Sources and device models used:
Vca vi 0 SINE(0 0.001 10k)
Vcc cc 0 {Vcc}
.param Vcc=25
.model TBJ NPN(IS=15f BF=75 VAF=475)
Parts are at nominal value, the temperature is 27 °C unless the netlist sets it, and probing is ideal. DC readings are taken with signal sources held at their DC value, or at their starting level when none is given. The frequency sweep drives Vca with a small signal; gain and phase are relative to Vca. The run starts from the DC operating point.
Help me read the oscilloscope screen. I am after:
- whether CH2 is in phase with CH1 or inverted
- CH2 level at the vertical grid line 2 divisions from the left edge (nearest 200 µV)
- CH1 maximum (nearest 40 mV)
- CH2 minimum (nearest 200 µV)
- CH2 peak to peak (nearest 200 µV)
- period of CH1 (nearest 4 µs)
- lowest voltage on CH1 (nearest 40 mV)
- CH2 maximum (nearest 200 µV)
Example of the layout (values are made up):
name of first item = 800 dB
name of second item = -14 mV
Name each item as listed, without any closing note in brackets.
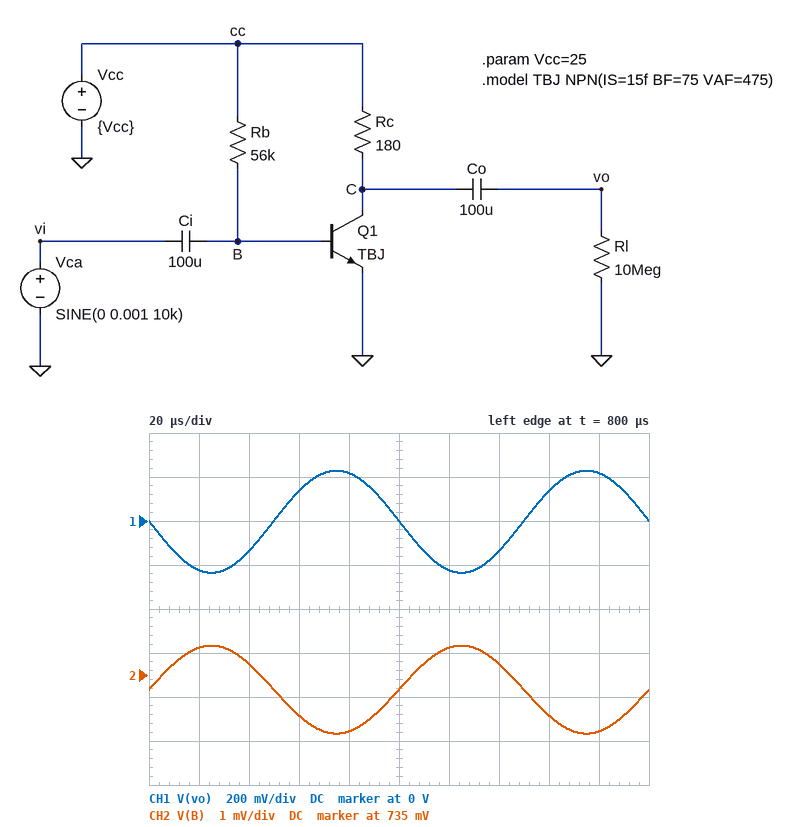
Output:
whether CH2 is in phase with CH1 or inverted = inverted
CH2 level at the vertical grid line 2 divisions from the left edge = 735.2 mV
CH1 maximum = 240 mV
CH2 minimum = 733.6 mV
CH2 peak to peak = 2.0 mV
period of CH1 = 100 µs
lowest voltage on CH1 = -240 mV
CH2 maximum = 735.6 mV
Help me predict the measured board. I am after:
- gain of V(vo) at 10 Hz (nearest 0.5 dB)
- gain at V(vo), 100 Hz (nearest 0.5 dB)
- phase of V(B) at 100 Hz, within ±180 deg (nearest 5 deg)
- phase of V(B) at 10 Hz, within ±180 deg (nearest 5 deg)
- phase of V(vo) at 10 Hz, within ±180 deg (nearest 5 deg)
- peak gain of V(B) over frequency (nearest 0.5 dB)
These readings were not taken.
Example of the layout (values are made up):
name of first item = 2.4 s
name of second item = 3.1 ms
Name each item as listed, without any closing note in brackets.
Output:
gain of V(vo) at 10 Hz = 38.0 dB
gain at V(vo), 100 Hz = 47.0 dB
phase of V(B) at 100 Hz, within ±180 deg = 15 deg
phase of V(B) at 10 Hz, within ±180 deg = 70 deg
phase of V(vo) at 10 Hz, within ±180 deg = -110 deg
peak gain of V(B) over frequency = 0 dB
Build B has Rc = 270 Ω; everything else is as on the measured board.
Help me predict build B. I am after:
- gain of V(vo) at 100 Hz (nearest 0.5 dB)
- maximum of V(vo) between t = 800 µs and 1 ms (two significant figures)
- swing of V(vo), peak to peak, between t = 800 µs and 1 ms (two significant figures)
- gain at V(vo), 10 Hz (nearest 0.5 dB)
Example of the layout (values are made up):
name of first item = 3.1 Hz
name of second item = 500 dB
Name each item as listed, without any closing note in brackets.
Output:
gain of V(vo) at 100 Hz = 50.5 dB
maximum of V(vo) between t = 800 µs and 1 ms = 340 mV
swing of V(vo), peak to peak, between t = 800 µs and 1 ms = 690 mV
gain at V(vo), 10 Hz = 41.5 dB
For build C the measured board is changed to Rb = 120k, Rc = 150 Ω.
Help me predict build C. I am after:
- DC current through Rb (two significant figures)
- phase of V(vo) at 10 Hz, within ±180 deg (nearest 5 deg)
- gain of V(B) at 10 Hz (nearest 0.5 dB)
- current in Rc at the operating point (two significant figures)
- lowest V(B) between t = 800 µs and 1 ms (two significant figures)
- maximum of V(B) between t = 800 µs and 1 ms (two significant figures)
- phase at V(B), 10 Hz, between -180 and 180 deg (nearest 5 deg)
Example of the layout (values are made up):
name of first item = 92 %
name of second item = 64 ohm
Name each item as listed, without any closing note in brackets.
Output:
DC current through Rb = 200 µA
phase of V(vo) at 10 Hz, within ±180 deg = -130 deg
gain of V(B) at 10 Hz = -4.0 dB
current in Rc at the operating point = 16 mA
lowest V(B) between t = 800 µs and 1 ms = 710 mV
maximum of V(B) between t = 800 µs and 1 ms = 720 mV
phase at V(B), 10 Hz, between -180 and 180 deg = 50 deg
